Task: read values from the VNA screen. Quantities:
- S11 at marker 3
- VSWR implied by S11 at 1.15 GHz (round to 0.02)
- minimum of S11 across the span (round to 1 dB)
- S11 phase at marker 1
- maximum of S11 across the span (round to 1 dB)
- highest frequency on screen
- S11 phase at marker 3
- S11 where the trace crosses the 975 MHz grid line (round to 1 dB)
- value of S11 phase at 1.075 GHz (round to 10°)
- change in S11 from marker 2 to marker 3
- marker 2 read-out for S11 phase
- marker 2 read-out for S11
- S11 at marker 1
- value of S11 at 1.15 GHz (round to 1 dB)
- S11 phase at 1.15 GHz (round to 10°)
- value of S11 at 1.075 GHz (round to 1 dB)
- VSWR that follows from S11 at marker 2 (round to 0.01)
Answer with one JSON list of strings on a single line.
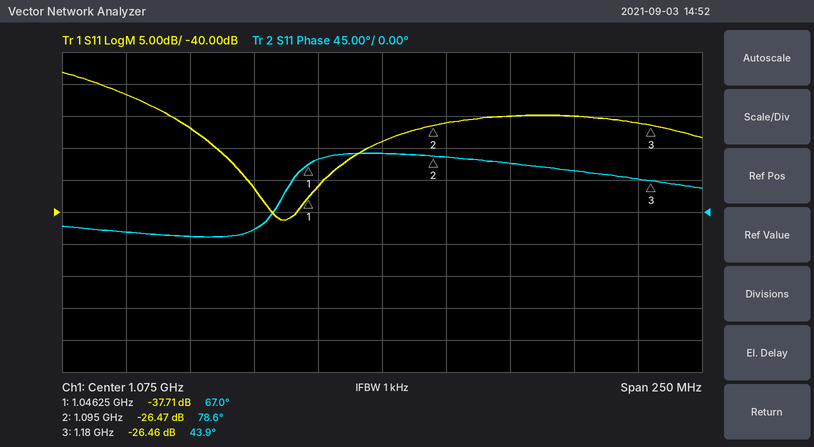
["-26.46 dB", "1.12", "-41 dB", "67.0°", "-18 dB", "1.2 GHz", "43.9°", "-22 dB", "80°", "0.01 dB", "78.6°", "-26.47 dB", "-37.71 dB", "-25 dB", "60°", "-29 dB", "1.10"]
